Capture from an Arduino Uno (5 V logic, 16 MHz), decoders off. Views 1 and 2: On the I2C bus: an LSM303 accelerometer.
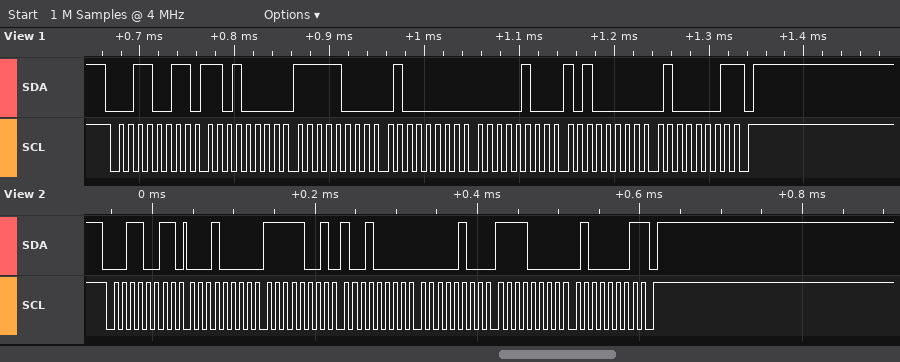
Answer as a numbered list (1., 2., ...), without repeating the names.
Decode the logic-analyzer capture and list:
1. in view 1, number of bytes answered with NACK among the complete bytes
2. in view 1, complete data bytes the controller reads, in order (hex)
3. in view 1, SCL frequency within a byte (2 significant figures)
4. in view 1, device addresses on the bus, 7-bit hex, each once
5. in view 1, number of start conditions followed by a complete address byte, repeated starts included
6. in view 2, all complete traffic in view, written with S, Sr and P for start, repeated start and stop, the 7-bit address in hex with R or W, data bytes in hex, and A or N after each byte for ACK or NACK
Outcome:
1. 1
2. D0 F8 40 04 A0 41
3. 100 kHz
4. 0x19
5. 1
6. S 19R A 10 A F9 A 90 A 04 A F0 A 41 N P
